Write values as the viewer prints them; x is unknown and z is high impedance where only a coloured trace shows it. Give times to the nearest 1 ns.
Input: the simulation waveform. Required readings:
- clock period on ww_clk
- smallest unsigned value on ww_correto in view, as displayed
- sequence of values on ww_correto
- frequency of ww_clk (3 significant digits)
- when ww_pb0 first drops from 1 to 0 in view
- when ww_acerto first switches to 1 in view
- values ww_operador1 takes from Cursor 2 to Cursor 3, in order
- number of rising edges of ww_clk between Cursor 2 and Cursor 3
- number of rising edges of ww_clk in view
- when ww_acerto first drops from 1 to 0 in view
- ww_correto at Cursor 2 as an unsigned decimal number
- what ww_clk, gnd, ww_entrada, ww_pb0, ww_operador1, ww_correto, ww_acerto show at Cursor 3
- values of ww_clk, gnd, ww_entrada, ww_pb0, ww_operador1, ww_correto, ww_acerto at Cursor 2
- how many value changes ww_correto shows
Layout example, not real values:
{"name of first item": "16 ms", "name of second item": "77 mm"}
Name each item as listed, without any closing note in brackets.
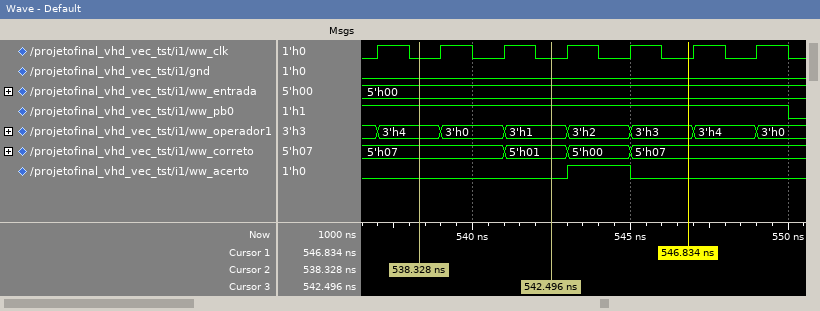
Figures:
{"clock period on ww_clk": "2 ns", "smallest unsigned value on ww_correto in view, as displayed": "5'h00", "sequence of values on ww_correto": "5'h07, 5'h01, 5'h00, 5'h07", "frequency of ww_clk": "500 MHz", "when ww_pb0 first drops from 1 to 0 in view": "550 ns", "when ww_acerto first switches to 1 in view": "543 ns", "values ww_operador1 takes from Cursor 2 to Cursor 3, in order": "3'h4, 3'h0, 3'h1", "number of rising edges of ww_clk between Cursor 2 and Cursor 3": "2", "number of rising edges of ww_clk in view": "7", "when ww_acerto first drops from 1 to 0 in view": "545 ns", "ww_correto at Cursor 2 as an unsigned decimal number": "7", "what ww_clk, gnd, ww_entrada, ww_pb0, ww_operador1, ww_correto, ww_acerto show at Cursor 3": "ww_clk=0, gnd=0, ww_entrada=5'h00, ww_pb0=1, ww_operador1=3'h1, ww_correto=5'h01, ww_acerto=0", "values of ww_clk, gnd, ww_entrada, ww_pb0, ww_operador1, ww_correto, ww_acerto at Cursor 2": "ww_clk=0, gnd=0, ww_entrada=5'h00, ww_pb0=1, ww_operador1=3'h4, ww_correto=5'h07, ww_acerto=0", "how many value changes ww_correto shows": "3"}
